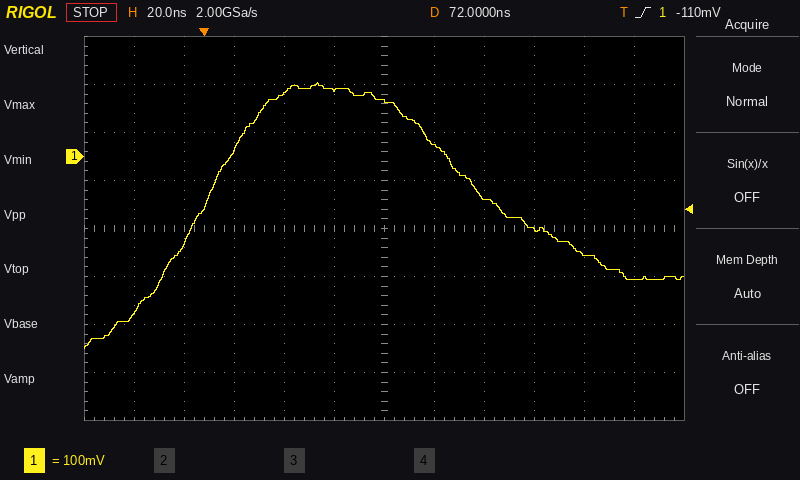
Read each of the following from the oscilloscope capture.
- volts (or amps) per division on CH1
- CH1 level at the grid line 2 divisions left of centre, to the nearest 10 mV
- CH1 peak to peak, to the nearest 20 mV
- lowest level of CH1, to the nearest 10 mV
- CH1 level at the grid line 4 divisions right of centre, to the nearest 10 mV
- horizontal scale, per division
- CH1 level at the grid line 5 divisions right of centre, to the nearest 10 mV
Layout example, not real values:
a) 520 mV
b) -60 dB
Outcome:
a) 100 mV
b) 130 mV
c) 560 mV
d) -400 mV
e) -200 mV
f) 20 ns
g) -260 mV
